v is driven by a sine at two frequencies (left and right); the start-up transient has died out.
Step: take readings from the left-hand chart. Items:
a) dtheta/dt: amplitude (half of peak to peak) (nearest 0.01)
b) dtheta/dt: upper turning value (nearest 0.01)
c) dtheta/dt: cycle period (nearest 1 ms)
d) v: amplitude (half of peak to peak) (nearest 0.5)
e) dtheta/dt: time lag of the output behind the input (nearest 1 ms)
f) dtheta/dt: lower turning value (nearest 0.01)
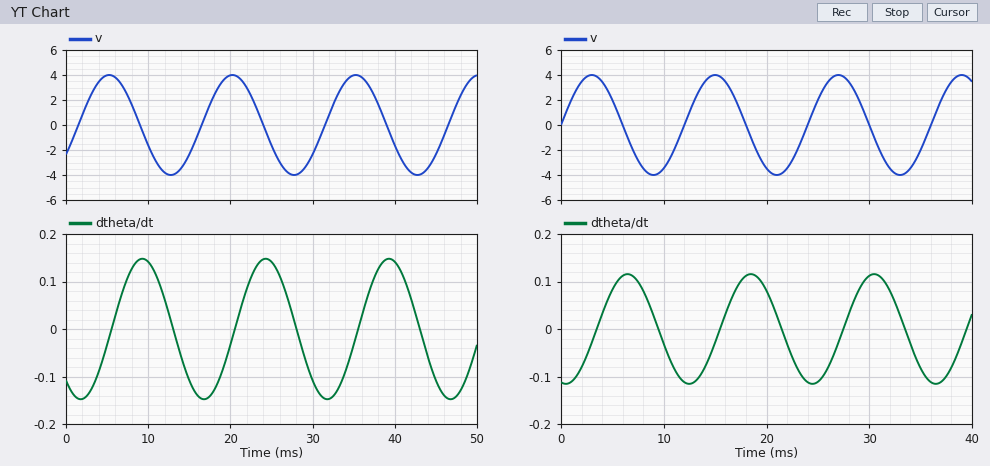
0.15
0.15
15 ms
4.0
4 ms
-0.15
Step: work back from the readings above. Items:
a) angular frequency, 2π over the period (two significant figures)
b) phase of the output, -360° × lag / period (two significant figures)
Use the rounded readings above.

0.42 rad/ms
-96°
